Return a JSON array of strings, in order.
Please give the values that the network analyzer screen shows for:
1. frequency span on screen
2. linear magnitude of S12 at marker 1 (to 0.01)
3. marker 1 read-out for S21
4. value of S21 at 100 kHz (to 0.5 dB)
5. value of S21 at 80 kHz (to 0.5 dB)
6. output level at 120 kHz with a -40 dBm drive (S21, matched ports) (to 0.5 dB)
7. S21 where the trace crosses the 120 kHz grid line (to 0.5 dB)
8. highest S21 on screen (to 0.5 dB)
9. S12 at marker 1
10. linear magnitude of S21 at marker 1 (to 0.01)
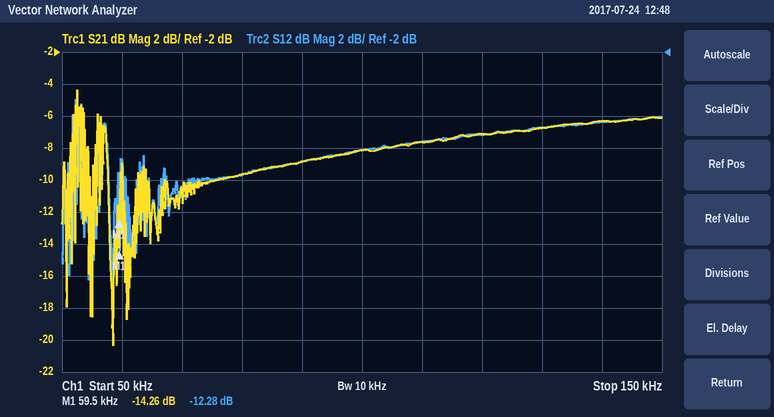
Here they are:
["100 kHz", "0.24", "-14.26 dB", "-8.0 dB", "-9.5 dB", "-47.0 dBm", "-7.0 dB", "-4.5 dB", "-12.28 dB", "0.19"]
